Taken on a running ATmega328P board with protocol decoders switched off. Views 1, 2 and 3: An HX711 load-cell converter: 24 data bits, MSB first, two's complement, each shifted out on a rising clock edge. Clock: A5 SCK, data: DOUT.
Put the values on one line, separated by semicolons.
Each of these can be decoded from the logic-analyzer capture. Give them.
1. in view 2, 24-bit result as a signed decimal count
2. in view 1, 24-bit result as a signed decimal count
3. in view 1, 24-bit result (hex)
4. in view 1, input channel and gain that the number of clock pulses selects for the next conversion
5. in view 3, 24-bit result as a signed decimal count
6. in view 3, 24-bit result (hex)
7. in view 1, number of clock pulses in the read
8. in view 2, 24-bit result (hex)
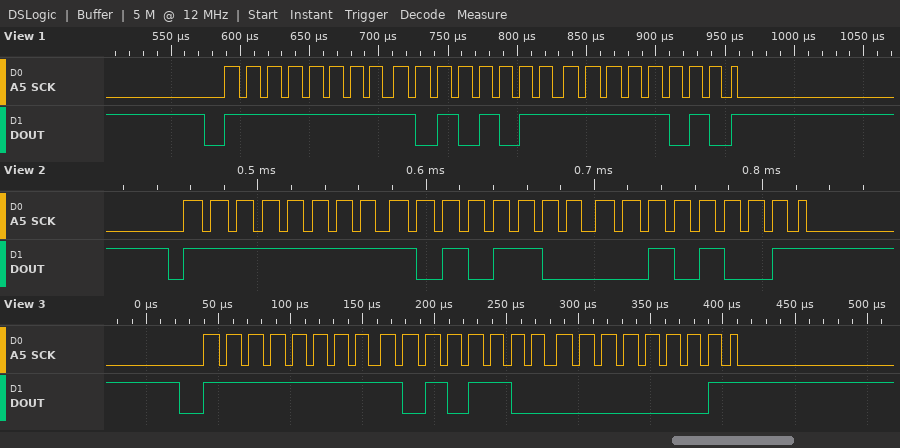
-21463; -21510; 0xFFABFA; channel A, gain 128; -21503; 0xFFAC01; 25; 0xFFAC29
